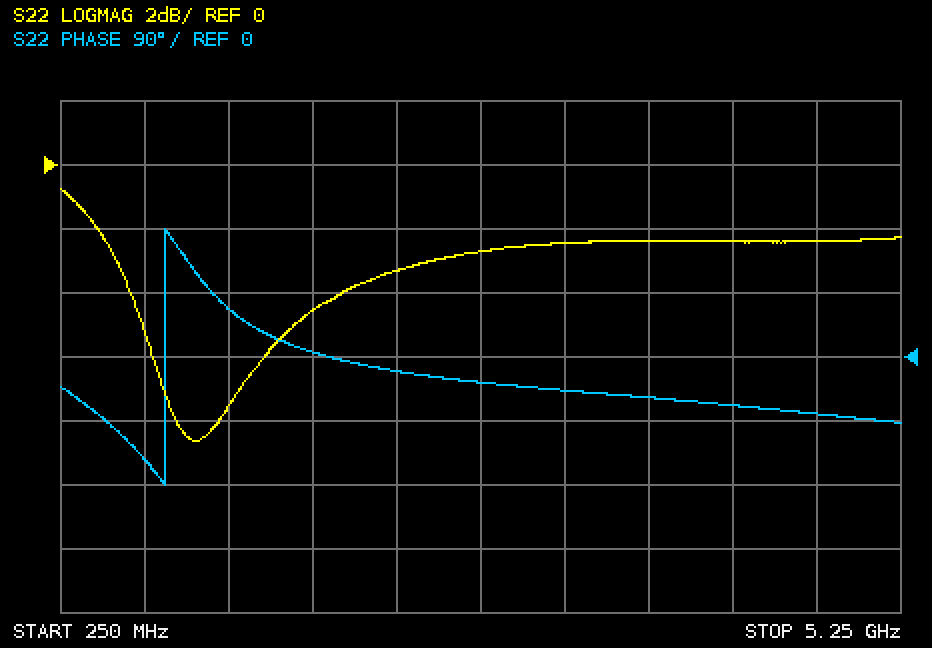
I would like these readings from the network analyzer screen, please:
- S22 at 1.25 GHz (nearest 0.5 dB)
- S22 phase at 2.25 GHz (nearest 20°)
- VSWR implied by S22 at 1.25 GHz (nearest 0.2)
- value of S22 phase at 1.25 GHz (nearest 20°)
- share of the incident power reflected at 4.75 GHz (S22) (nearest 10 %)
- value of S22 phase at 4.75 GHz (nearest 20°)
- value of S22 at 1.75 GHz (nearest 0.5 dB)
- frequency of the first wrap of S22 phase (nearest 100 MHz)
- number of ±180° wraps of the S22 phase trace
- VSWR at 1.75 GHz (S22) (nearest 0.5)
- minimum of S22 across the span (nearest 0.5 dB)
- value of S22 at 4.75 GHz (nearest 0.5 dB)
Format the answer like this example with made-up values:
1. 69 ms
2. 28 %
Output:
1. -7.5 dB
2. -20°
3. 2.4
4. 60°
5. 60 %
6. -80°
7. -4.5 dB
8. 900 MHz
9. 1
10. 4.0
11. -8.5 dB
12. -2.5 dB
